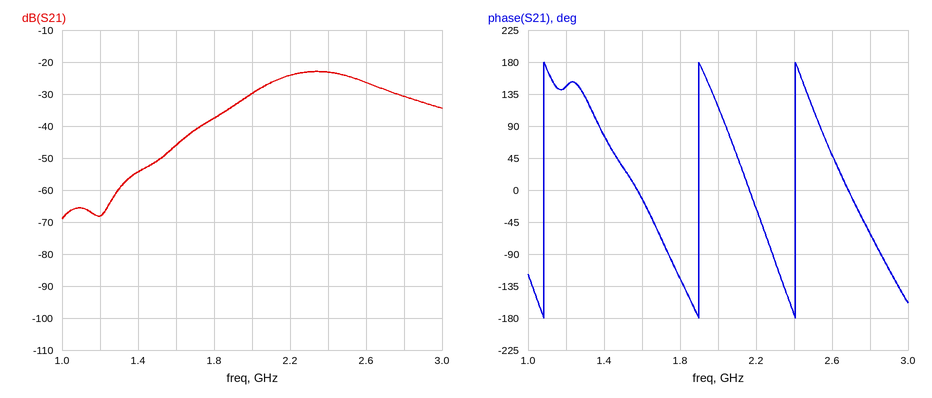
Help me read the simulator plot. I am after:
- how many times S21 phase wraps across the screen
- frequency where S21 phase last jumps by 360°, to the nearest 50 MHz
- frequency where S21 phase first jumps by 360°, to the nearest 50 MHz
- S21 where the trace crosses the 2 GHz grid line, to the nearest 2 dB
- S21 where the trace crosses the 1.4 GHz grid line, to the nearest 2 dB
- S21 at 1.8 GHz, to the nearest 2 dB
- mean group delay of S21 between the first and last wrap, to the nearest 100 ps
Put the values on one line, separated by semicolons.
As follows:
3; 2.40 GHz; 1.10 GHz; -30 dB; -54 dB; -38 dB; 1.5 ns
